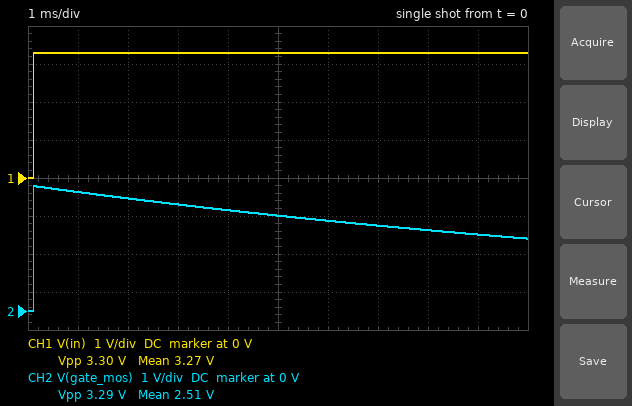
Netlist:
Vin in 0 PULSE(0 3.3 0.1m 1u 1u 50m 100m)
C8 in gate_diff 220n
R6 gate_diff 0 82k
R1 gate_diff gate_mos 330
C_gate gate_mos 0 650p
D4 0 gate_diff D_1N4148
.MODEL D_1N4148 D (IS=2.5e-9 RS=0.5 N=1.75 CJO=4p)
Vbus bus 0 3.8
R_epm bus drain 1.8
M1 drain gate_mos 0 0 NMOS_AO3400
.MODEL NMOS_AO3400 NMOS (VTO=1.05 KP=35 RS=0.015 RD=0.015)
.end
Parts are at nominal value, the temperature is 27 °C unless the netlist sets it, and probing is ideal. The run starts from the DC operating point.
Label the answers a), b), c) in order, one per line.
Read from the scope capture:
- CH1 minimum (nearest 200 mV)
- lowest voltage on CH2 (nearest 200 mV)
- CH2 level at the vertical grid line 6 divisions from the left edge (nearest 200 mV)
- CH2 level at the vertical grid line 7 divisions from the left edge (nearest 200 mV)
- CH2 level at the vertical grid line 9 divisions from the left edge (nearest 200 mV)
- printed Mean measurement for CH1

a) 0 V
b) 0 V
c) 2.4 V
d) 2.2 V
e) 2.0 V
f) 3.27 V
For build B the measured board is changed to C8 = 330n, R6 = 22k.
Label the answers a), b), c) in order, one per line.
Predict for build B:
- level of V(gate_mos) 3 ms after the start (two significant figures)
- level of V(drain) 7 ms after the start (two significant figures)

a) 2.2 V
b) 2.4 V
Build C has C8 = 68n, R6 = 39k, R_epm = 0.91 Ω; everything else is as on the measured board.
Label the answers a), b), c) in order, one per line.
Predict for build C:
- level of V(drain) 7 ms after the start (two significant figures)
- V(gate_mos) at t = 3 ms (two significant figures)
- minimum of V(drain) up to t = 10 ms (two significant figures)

a) 3.8 V
b) 1.1 V
c) 170 mV
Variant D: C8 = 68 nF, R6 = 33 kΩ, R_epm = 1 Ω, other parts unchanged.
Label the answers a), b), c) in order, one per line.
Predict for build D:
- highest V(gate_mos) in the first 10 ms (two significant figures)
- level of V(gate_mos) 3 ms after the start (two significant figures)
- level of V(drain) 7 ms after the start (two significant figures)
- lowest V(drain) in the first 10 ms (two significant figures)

a) 3.3 V
b) 910 mV
c) 3.8 V
d) 160 mV
